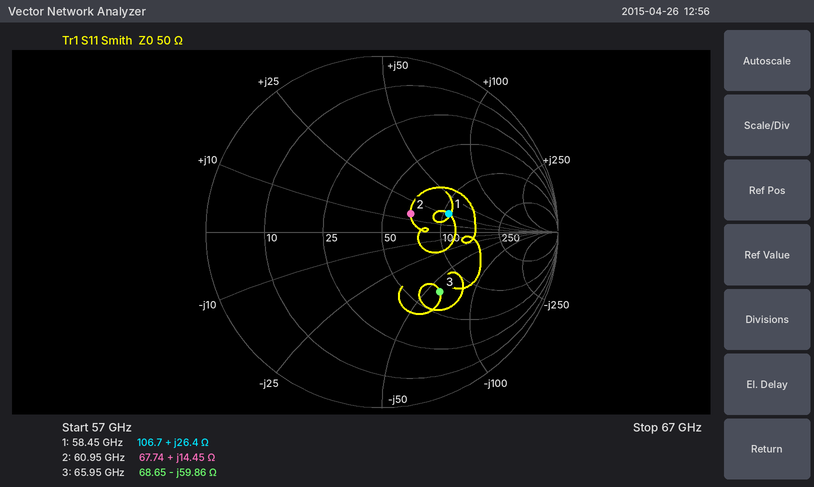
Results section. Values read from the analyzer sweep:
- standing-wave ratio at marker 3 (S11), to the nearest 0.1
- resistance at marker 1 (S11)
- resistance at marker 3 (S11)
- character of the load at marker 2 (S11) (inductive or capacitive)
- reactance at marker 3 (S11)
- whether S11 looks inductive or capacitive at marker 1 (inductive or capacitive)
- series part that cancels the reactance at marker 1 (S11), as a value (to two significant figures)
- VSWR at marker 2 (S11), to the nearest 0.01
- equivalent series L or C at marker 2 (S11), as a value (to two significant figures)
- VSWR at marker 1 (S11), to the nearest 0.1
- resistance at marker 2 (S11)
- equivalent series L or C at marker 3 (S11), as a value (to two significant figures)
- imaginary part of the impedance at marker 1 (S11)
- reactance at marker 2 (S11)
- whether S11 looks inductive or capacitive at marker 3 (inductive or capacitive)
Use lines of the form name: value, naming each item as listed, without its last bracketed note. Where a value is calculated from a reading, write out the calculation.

standing-wave ratio at marker 3 (S11), to the nearest 0.1: 2.8
resistance at marker 1: 106.7 Ω
resistance at marker 3: 68.65 Ω
character of the load at marker 2 (S11): inductive
reactance at marker 3: -59.86 Ω
whether S11 looks inductive or capacitive at marker 1: inductive
series part that cancels the reactance at marker 1 (S11), as a value: C = 1/(2π × 58.45 GHz × 26.4 Ω) ≈ 103 fF, so 100 fF to two significant figures
VSWR at marker 2 (S11), to the nearest 0.01: 1.48
equivalent series L or C at marker 2 (S11), as a value: L = 14.45 Ω/(2π × 60.95 GHz) ≈ 38 pH
VSWR at marker 1 (S11), to the nearest 0.1: 2.3
resistance at marker 2: 67.74 Ω
equivalent series L or C at marker 3 (S11), as a value: C = 1/(2π × 65.95 GHz × 59.86 Ω) ≈ 40 fF
imaginary part of the impedance at marker 1: +26.4 Ω
reactance at marker 2: +14.45 Ω
whether S11 looks inductive or capacitive at marker 3: capacitive
